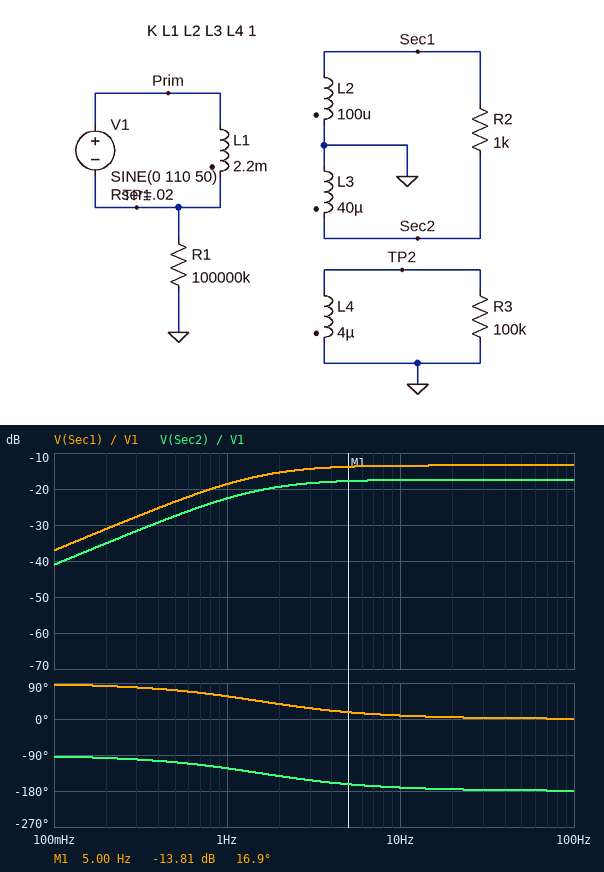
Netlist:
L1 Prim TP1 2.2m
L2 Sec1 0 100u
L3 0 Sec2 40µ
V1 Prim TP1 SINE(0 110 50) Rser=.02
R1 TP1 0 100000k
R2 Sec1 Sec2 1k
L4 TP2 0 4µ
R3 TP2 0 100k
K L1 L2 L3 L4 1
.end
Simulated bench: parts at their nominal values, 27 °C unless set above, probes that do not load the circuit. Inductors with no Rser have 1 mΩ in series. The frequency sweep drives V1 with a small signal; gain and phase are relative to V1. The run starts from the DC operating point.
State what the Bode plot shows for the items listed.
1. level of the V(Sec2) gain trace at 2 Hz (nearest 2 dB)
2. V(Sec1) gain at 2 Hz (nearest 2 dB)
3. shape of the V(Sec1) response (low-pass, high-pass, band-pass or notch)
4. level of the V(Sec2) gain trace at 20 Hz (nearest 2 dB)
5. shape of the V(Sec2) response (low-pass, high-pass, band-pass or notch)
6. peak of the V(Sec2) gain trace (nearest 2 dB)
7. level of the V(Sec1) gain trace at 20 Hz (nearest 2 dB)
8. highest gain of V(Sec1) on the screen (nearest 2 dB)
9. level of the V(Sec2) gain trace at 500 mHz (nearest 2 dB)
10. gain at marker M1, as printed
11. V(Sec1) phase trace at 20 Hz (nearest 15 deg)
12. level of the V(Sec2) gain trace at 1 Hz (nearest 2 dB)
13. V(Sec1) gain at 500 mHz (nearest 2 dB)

-20 dB
-16 dB
high-pass
-18 dB
high-pass
-18 dB
-14 dB
-14 dB
-28 dB
-13.81 dB
0 deg
-22 dB
-24 dB
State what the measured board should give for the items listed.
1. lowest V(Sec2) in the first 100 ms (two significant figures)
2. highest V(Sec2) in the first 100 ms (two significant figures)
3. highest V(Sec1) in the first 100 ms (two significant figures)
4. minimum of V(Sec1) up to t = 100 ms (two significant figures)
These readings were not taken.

-15 V
15 V
23 V
-24 V
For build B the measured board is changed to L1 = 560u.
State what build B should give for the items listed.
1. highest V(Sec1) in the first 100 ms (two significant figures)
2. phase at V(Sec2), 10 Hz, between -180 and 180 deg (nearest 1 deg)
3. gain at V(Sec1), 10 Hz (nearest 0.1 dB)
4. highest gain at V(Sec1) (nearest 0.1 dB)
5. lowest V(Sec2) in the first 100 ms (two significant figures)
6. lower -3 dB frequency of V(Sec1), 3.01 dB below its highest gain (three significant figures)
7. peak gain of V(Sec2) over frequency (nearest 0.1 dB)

46 V
-149 deg
-8.8 dB
-7.5 dB
-29 V
5.97 Hz
-11.5 dB
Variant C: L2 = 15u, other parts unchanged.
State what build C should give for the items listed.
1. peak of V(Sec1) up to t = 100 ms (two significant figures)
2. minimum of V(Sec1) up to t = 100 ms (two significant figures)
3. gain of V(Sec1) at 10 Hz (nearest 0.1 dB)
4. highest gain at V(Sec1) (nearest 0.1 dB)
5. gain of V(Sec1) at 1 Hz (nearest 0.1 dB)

9.0 V
-9.3 V
-21.8 dB
-21.7 dB
-26.9 dB
